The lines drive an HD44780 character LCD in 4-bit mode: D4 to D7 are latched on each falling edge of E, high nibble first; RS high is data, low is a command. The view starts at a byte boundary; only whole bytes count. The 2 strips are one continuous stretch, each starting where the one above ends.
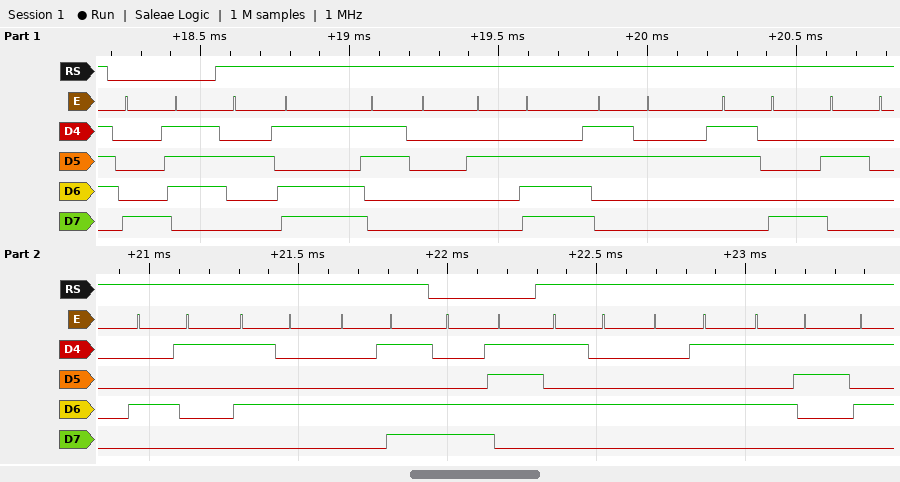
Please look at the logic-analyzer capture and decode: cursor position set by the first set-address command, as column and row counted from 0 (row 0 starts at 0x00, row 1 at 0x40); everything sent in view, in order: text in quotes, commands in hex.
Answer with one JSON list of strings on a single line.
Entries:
["column 7, row 0", "0x87 \"-0.28 ATM\" 0xC7 \"TES\""]
